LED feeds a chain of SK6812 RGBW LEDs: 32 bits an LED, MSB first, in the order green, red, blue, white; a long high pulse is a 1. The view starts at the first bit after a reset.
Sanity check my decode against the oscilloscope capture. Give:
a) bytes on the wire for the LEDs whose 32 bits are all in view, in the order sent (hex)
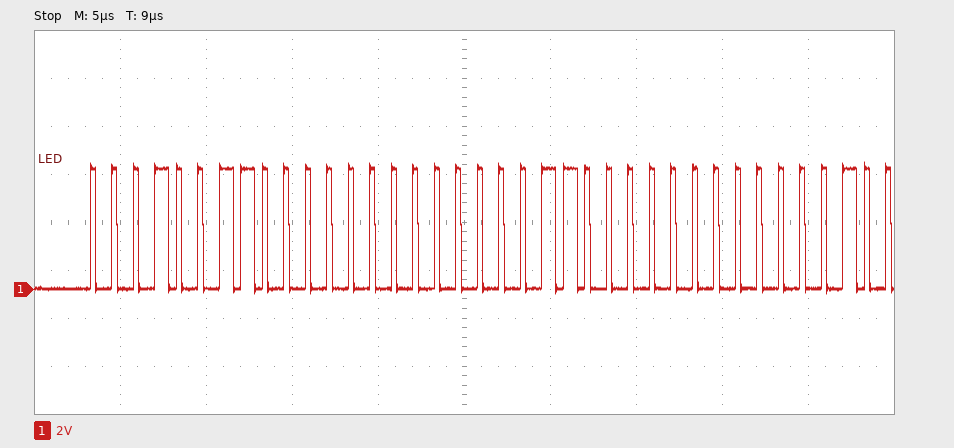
13 00 06 00
